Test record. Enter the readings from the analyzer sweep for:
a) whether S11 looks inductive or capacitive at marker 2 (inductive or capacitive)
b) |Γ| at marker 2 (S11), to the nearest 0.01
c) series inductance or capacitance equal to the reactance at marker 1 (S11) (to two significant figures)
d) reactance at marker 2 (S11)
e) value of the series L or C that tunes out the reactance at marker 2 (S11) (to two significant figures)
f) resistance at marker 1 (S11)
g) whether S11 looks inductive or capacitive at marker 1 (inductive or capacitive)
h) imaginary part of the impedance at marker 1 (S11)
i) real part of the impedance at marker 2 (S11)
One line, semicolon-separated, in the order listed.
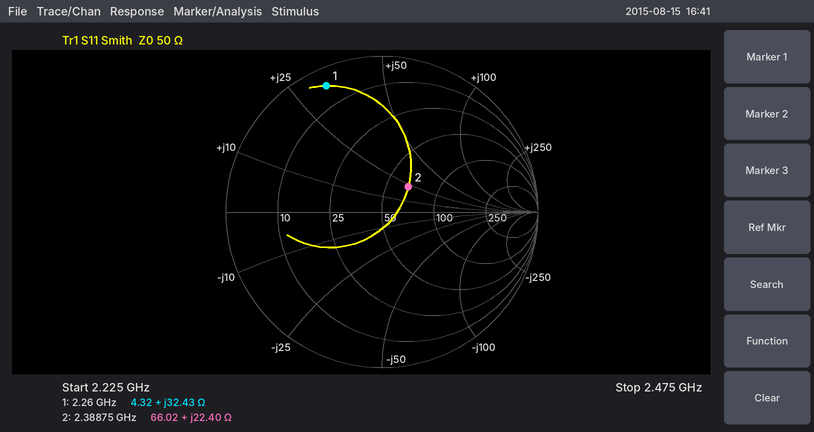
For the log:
inductive; 0.23; 2.3 nH; +22.40 Ω; 3.0 pF; 4.32 Ω; inductive; +32.43 Ω; 66.02 Ω
